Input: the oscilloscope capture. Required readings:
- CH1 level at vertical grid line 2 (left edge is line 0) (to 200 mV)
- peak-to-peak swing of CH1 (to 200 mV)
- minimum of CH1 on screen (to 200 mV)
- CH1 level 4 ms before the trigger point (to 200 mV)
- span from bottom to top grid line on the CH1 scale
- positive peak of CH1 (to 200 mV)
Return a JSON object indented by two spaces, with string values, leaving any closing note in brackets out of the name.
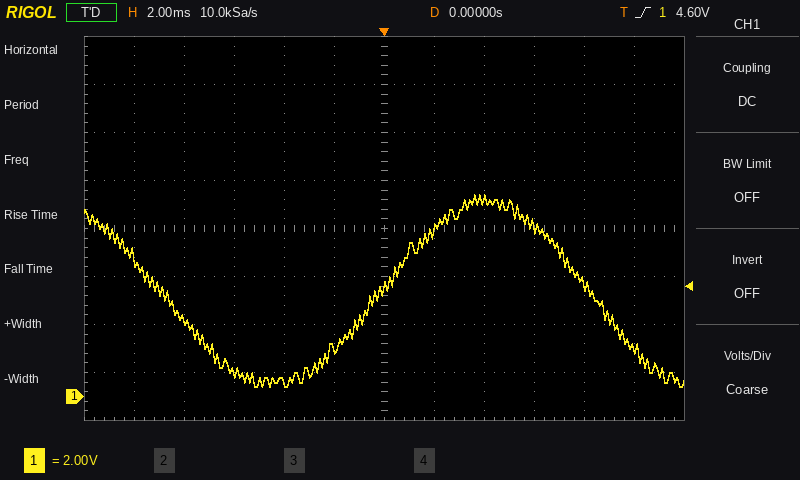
{
  "CH1 level at vertical grid line 2 (left edge is line 0)": "3.2 V",
  "peak-to-peak swing of CH1": "8.0 V",
  "minimum of CH1 on screen": "400 mV",
  "CH1 level 4 ms before the trigger point": "600 mV",
  "span from bottom to top grid line on the CH1 scale": "16 V",
  "positive peak of CH1": "8.4 V"
}
